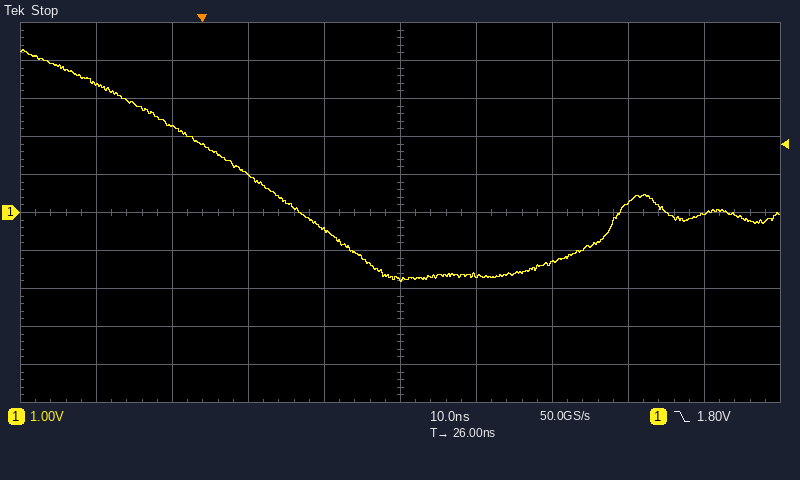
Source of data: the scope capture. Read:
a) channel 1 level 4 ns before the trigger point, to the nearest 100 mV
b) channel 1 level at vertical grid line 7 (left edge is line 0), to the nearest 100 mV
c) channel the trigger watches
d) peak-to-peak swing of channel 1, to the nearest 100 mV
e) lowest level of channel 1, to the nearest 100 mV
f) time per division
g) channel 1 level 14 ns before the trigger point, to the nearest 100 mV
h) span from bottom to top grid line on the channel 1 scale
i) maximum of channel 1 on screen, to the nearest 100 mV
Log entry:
2.3 V
-1.3 V
channel 1
6.1 V
-1.8 V
10 ns
3.4 V
10 V
4.3 V
